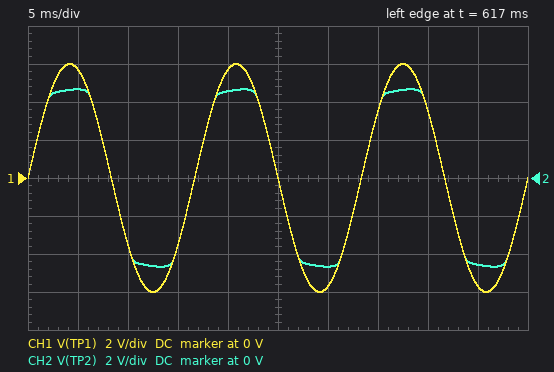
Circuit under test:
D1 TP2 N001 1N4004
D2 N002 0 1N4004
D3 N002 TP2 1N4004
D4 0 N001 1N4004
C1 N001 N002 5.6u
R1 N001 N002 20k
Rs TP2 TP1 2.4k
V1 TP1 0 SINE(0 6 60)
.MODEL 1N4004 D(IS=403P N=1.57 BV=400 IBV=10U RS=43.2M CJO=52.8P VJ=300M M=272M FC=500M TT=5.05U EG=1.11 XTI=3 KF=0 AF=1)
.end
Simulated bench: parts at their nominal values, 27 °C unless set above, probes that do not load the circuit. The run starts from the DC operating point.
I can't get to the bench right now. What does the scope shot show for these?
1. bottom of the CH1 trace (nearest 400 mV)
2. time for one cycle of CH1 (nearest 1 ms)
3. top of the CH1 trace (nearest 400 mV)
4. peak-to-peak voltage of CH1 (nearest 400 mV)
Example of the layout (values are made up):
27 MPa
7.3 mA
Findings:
-6.0 V
17 ms
6.0 V
12.0 V
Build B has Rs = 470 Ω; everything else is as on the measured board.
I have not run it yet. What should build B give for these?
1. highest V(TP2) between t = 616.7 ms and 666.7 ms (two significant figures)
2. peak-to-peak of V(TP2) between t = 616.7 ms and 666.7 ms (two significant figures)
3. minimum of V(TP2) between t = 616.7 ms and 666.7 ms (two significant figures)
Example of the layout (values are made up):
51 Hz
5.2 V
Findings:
5.5 V
11 V
-5.5 V
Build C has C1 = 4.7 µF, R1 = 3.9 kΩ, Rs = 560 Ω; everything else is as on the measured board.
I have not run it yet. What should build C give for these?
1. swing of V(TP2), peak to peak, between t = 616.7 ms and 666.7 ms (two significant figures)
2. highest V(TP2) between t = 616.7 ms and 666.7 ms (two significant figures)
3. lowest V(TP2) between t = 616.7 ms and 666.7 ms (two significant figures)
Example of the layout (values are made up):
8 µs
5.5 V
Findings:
9.6 V
4.8 V
-4.8 V
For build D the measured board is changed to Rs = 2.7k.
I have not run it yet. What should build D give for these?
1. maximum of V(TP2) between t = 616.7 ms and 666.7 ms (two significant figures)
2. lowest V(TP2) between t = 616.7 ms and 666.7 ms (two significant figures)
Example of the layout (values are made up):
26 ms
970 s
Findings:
4.6 V
-4.6 V
